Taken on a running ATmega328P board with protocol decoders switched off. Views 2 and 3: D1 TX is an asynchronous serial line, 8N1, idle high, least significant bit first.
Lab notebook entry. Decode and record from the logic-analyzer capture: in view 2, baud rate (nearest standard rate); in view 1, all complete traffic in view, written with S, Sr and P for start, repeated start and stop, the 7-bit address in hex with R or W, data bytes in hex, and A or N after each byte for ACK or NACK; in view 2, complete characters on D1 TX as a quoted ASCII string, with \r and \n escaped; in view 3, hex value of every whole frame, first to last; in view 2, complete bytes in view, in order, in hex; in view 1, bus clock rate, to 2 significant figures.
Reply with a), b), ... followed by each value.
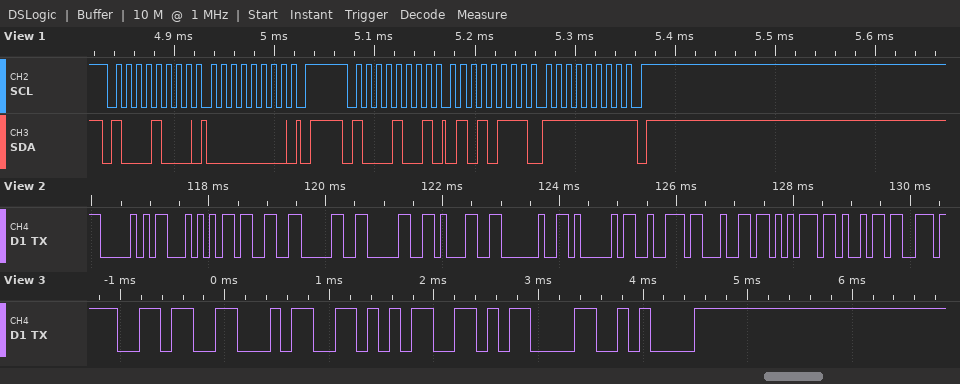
a) 9600 baud
b) S 44W A 00 A P S 44R A 57 A FF N P
c) "PT3001 Ardui"
d) 0x36 0x34 0x35 0x0D 0x0A
e) 50 54 33 30 30 31 20 41 72 64 75 69
f) 100 kHz
